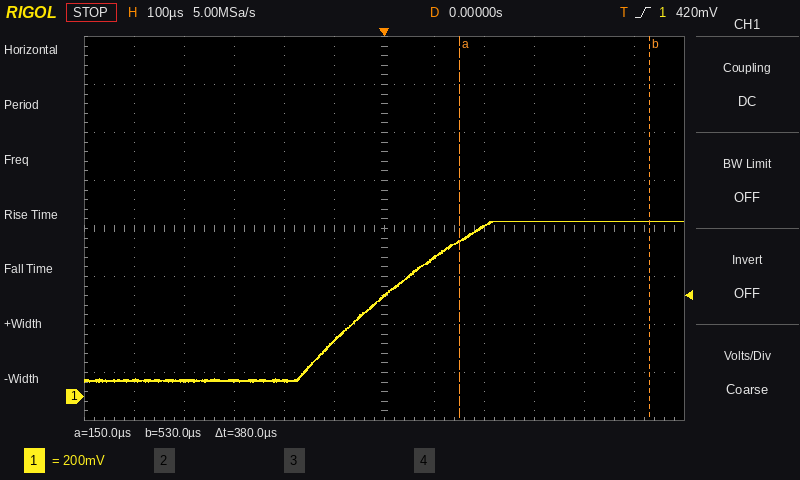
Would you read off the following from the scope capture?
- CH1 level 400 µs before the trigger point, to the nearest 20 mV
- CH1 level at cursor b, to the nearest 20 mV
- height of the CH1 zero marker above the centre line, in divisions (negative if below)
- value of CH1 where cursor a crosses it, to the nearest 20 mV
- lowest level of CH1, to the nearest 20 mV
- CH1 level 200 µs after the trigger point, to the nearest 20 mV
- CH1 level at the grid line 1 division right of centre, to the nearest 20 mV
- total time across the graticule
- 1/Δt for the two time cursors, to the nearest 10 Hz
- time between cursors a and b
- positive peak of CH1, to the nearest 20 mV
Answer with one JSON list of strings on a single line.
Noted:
["60 mV", "720 mV", "-3.5 div", "640 mV", "60 mV", "700 mV", "580 mV", "1.2 ms", "2.63 kHz", "380 µs", "720 mV"]
